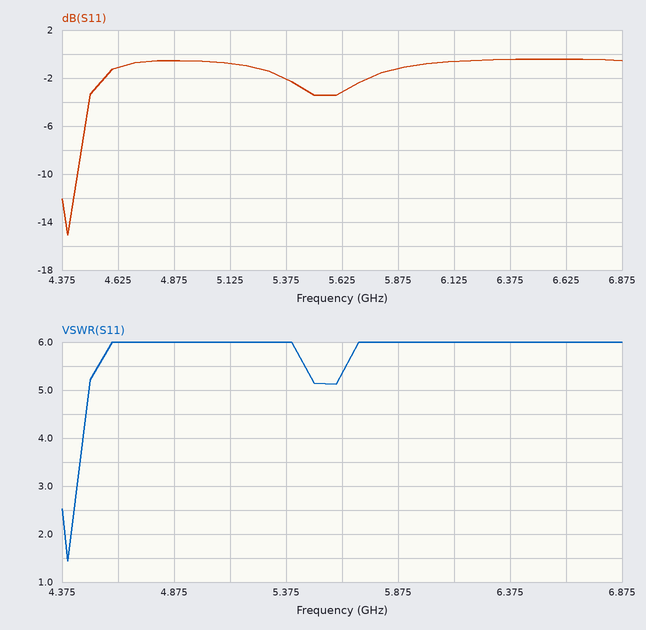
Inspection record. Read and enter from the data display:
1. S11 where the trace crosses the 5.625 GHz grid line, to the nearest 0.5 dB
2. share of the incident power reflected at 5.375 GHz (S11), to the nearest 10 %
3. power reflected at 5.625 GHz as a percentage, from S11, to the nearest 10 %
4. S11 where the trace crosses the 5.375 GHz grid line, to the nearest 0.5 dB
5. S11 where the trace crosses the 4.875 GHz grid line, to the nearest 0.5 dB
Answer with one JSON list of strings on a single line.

["-3.0 dB", "60 %", "50 %", "-2.0 dB", "-0.5 dB"]
